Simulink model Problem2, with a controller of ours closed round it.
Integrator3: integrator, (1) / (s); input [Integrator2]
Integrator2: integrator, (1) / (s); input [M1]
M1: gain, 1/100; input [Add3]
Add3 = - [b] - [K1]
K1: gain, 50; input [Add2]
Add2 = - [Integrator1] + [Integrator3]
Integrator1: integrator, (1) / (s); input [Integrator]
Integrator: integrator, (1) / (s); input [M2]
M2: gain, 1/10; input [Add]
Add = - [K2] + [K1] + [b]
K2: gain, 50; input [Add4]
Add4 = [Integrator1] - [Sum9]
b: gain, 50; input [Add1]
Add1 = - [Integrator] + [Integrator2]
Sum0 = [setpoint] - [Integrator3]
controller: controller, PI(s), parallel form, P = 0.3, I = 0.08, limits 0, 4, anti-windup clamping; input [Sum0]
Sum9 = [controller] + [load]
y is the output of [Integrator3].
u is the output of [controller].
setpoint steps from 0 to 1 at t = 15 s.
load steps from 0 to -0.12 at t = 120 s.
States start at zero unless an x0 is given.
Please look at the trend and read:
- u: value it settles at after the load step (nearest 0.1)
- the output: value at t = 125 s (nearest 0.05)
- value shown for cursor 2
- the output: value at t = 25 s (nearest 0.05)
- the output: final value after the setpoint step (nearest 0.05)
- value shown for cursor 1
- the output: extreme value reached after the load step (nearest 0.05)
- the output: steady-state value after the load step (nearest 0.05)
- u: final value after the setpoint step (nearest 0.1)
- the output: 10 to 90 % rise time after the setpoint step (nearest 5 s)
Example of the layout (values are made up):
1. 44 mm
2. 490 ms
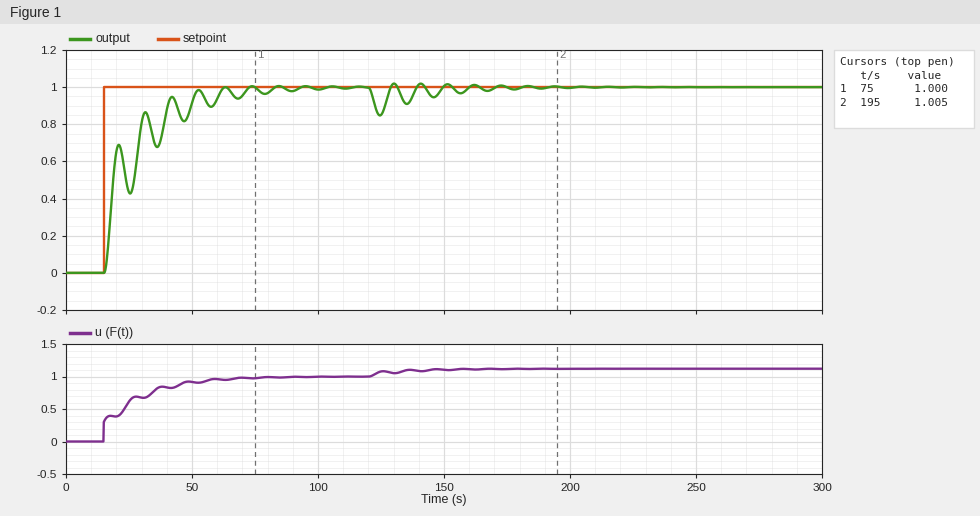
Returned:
1. 1.1
2. 0.85
3. 1.005
4. 0.45
5. 1.00
6. 1.000
7. 0.85
8. 1.00
9. 1.0
10. 25 s
